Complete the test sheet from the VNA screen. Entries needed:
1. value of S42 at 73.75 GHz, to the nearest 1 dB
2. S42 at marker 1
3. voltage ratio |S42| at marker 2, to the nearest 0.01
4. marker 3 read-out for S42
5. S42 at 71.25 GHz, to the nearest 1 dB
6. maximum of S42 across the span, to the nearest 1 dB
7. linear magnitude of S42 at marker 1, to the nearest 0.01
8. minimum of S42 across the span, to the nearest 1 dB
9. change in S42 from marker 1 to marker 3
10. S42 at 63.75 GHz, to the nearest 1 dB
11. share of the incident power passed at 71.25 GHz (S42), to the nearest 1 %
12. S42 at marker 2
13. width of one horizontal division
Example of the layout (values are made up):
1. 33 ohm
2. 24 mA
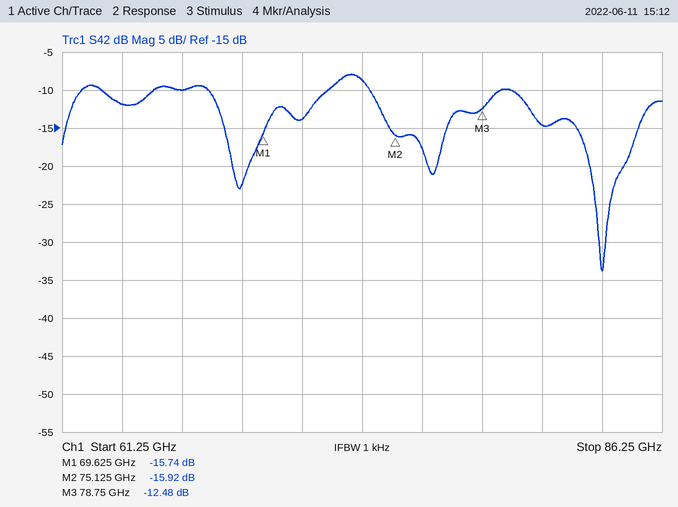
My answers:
1. -9 dB
2. -15.74 dB
3. 0.16
4. -12.48 dB
5. -14 dB
6. -8 dB
7. 0.16
8. -34 dB
9. 3.26 dB
10. -12 dB
11. 4 %
12. -15.92 dB
13. 2.5 GHz
